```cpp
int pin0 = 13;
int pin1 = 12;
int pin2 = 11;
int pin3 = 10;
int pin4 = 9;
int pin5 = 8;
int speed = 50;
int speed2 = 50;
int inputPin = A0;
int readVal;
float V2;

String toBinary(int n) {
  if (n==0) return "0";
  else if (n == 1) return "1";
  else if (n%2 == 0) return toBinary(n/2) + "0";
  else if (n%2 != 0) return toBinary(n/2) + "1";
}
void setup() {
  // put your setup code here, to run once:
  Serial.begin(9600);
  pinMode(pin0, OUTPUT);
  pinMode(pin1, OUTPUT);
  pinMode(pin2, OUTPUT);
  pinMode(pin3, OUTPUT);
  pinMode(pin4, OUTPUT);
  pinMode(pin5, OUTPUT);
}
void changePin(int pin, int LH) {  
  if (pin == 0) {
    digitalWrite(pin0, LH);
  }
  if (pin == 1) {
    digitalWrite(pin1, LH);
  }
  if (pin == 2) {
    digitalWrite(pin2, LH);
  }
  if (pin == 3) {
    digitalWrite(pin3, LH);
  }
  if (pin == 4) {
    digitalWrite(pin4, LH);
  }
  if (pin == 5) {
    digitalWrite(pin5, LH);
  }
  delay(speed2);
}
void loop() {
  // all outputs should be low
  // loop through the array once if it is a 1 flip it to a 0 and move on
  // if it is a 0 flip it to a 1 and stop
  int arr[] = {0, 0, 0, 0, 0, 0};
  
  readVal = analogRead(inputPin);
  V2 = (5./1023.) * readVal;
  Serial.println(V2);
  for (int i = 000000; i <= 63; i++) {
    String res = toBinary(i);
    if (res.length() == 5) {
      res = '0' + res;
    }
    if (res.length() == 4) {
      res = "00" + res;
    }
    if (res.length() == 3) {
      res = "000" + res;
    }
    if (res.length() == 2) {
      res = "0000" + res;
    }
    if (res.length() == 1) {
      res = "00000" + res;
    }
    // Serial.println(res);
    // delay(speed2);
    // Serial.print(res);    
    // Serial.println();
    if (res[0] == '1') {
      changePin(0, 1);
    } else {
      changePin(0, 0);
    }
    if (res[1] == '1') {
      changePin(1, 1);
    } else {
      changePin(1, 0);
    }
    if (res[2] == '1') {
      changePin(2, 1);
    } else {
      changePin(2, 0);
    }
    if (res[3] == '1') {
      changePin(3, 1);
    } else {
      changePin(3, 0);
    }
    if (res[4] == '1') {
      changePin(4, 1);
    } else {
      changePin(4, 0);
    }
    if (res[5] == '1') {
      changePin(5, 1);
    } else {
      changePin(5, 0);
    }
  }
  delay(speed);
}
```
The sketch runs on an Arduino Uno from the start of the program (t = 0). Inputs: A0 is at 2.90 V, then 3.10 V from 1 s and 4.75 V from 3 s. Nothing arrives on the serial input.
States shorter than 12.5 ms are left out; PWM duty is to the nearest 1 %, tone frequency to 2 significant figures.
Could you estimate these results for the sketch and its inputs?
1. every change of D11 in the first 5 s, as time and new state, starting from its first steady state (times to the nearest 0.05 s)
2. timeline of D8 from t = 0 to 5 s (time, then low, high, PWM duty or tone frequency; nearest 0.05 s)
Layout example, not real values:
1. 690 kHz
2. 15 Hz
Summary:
1. 0 s low; 2.5 s high; 4.9 s low
2. 0 s low; 0.55 s high; 0.85 s low; 1.15 s high; 1.45 s low; 1.75 s high; 2.05 s low; 2.35 s high; 2.65 s low; 2.95 s high; 3.25 s low; 3.55 s high; 3.85 s low; 4.15 s high; 4.45 s low; 4.75 s high
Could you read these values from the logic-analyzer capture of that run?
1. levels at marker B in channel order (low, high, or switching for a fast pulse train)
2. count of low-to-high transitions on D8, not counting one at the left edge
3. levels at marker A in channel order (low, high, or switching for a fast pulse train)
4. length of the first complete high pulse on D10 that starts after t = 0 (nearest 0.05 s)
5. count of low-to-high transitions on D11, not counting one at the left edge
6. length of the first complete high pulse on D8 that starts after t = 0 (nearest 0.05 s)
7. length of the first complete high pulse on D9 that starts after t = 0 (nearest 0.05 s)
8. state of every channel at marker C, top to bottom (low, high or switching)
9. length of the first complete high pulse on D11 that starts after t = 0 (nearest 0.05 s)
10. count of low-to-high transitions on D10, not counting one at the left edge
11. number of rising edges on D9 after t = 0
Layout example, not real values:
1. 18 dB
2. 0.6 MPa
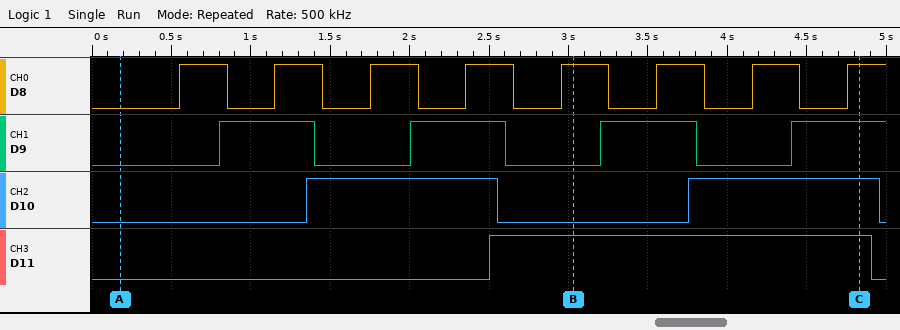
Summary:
1. D8 high, D9 low, D10 low, D11 high
2. 8
3. D8 low, D9 low, D10 low, D11 low
4. 1.20 s
5. 1
6. 0.30 s
7. 0.60 s
8. D8 high, D9 high, D10 high, D11 high
9. 2.40 s
10. 2
11. 4
